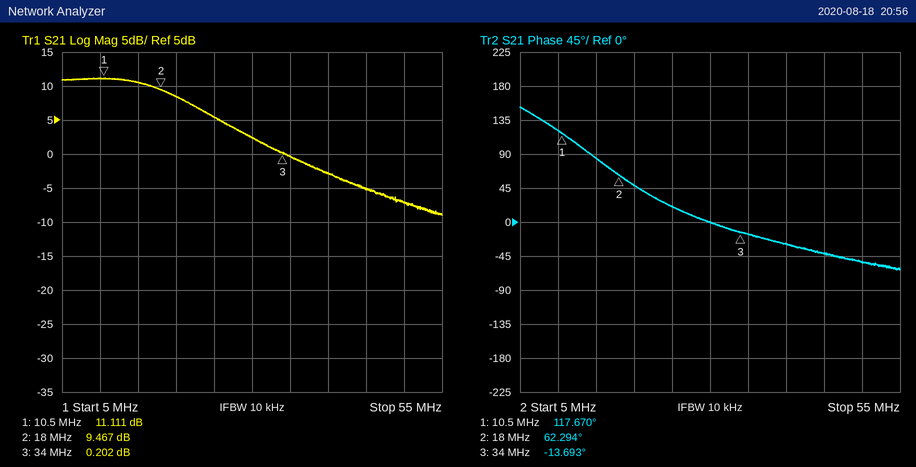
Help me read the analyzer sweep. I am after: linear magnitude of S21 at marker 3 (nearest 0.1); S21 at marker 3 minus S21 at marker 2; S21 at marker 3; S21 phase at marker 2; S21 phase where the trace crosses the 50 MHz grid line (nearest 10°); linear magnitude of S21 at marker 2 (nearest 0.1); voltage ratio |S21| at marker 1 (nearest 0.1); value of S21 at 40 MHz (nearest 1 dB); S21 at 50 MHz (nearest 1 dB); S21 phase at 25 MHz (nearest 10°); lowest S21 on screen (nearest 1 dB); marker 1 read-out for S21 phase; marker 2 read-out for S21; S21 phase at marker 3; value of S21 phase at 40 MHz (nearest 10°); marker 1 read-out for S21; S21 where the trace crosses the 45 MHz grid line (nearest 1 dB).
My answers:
1.0
-9.265 dB
0.202 dB
62.294°
-50°
3.0
3.6
-3 dB
-7 dB
20°
-9 dB
117.670°
9.467 dB
-13.693°
-30°
11.111 dB
-5 dB
